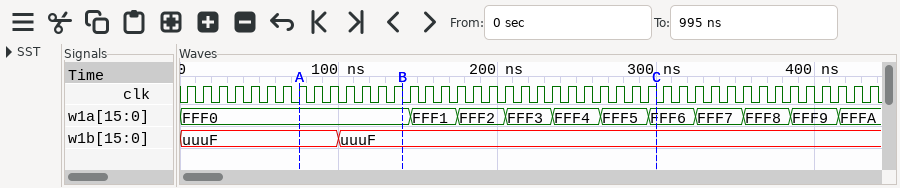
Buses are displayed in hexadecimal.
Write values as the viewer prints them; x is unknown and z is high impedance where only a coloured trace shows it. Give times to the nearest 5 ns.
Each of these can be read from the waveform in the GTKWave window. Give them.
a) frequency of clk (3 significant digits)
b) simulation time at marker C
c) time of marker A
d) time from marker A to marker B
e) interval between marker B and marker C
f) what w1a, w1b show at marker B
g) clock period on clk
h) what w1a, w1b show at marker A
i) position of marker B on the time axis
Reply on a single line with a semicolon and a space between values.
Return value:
100 MHz; 300 ns; 75 ns; 65 ns; 160 ns; w1a=FFF0, w1b=uuuF; 10 ns; w1a=FFF0, w1b=uuuF; 140 ns
